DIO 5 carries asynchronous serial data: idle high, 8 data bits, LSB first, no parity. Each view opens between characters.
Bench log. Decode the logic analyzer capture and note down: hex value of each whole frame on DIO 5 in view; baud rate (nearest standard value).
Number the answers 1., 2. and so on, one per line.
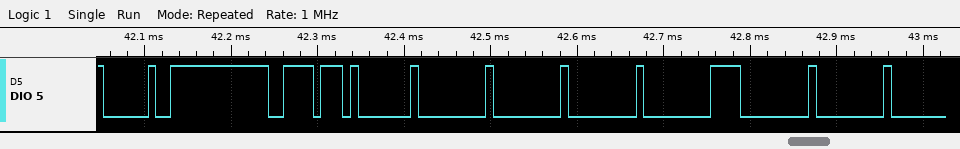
1. 20, DE, 01, 00, 00, 00, 00, 00, 00
2. 115200 baud
